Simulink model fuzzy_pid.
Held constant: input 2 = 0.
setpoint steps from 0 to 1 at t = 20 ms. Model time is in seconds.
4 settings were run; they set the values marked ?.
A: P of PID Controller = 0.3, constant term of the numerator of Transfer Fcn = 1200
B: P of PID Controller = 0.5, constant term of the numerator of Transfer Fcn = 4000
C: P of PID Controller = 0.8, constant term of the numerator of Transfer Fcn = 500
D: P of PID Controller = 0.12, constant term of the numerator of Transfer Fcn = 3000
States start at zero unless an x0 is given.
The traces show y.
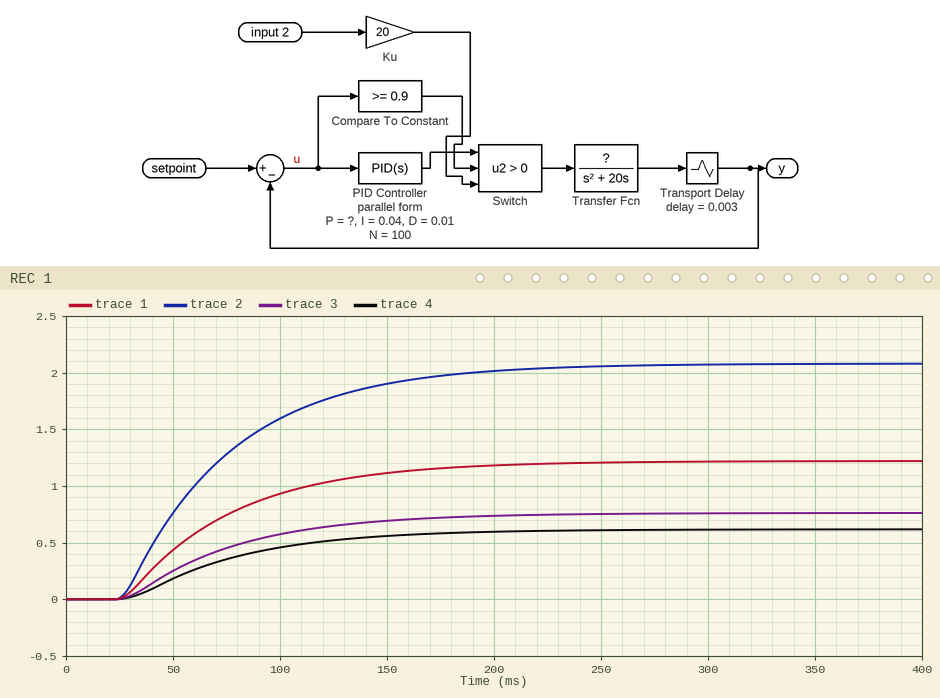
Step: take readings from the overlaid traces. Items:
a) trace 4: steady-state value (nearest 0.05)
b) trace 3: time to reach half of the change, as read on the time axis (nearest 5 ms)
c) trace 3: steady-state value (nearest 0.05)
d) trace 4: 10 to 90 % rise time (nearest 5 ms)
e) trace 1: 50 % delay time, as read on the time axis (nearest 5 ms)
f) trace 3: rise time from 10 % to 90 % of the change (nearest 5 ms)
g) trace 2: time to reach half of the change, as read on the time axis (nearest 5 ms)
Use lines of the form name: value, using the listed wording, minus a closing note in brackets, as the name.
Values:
trace 4: steady-state value: 0.60
trace 3: time to reach half of the change, as read on the time axis: 65 ms
trace 3: steady-state value: 0.75
trace 4: 10 to 90 % rise time: 110 ms
trace 1: 50 % delay time, as read on the time axis: 65 ms
trace 3: rise time from 10 % to 90 % of the change: 110 ms
trace 2: time to reach half of the change, as read on the time axis: 60 ms
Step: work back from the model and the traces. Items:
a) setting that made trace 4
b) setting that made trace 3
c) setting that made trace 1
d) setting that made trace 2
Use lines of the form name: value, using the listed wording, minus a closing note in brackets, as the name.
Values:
setting that made trace 4: C
setting that made trace 3: A
setting that made trace 1: D
setting that made trace 2: B
